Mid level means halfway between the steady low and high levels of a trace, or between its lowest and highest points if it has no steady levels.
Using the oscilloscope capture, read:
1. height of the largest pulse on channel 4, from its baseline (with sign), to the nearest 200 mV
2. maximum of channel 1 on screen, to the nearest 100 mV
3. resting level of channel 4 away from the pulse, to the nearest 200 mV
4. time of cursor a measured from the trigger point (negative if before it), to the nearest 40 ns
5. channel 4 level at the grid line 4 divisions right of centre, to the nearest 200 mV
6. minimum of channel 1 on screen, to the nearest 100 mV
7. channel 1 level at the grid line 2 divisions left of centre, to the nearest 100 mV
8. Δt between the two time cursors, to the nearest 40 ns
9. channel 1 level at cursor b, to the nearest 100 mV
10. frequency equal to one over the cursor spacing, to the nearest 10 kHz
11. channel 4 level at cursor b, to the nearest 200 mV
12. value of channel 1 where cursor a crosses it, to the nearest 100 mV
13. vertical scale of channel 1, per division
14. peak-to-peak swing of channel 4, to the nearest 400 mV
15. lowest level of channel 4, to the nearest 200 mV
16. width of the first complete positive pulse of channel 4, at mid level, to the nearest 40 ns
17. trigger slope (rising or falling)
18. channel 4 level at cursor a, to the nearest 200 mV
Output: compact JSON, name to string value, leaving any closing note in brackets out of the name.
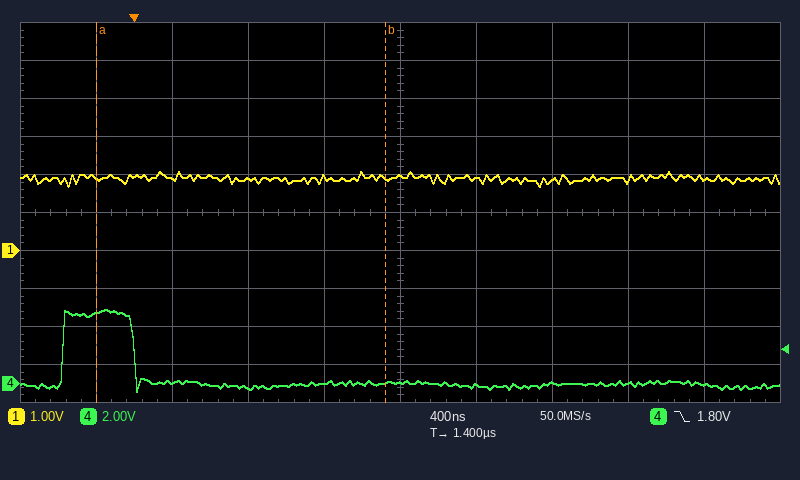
{"height of the largest pulse on channel 4, from its baseline (with sign), to the nearest 200 mV": "+4.0 V", "maximum of channel 1 on screen, to the nearest 100 mV": "2.1 V", "resting level of channel 4 away from the pulse, to the nearest 200 mV": "0.0 V", "time of cursor a measured from the trigger point (negative if before it), to the nearest 40 ns": "-200 ns", "channel 4 level at the grid line 4 divisions right of centre, to the nearest 200 mV": "0.0 V", "minimum of channel 1 on screen, to the nearest 100 mV": "1.7 V", "channel 1 level at the grid line 2 divisions left of centre, to the nearest 100 mV": "1.9 V", "Δt between the two time cursors, to the nearest 40 ns": "1.52 µs", "channel 1 level at cursor b, to the nearest 100 mV": "1.9 V", "frequency equal to one over the cursor spacing, to the nearest 10 kHz": "660 kHz", "channel 4 level at cursor b, to the nearest 200 mV": "0.0 V", "value of channel 1 where cursor a crosses it, to the nearest 100 mV": "1.9 V", "vertical scale of channel 1, per division": "1 V", "peak-to-peak swing of channel 4, to the nearest 400 mV": "4.4 V", "lowest level of channel 4, to the nearest 200 mV": "-400 mV", "width of the first complete positive pulse of channel 4, at mid level, to the nearest 40 ns": "360 ns", "trigger slope": "falling", "channel 4 level at cursor a, to the nearest 200 mV": "3.8 V"}
